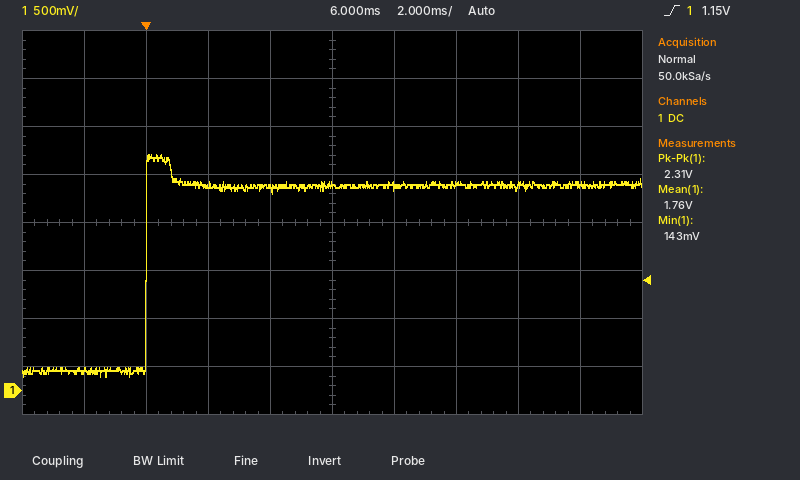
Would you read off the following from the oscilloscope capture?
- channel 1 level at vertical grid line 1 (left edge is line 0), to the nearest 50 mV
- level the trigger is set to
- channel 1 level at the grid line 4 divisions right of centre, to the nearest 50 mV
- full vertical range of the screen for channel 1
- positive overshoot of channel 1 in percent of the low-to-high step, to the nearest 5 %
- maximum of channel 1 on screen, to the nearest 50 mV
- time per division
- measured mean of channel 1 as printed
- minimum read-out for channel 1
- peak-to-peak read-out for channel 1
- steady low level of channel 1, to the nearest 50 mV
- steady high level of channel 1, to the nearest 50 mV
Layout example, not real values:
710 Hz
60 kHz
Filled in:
200 mV
1.15 V
2.15 V
4 V
15 %
2.45 V
2 ms
1.76 V
143 mV
2.31 V
200 mV
2.15 V
